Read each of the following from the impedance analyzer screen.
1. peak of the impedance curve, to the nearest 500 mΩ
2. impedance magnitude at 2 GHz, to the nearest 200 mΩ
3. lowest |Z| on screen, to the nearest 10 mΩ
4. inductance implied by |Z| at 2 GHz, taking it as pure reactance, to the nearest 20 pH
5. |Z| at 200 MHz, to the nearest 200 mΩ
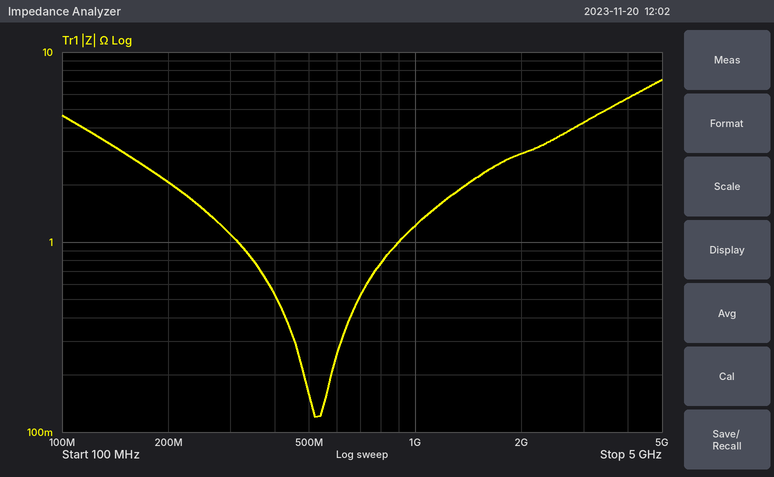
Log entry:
7.0 Ω
3.0 Ω
120 mΩ
240 pH
2.0 Ω
